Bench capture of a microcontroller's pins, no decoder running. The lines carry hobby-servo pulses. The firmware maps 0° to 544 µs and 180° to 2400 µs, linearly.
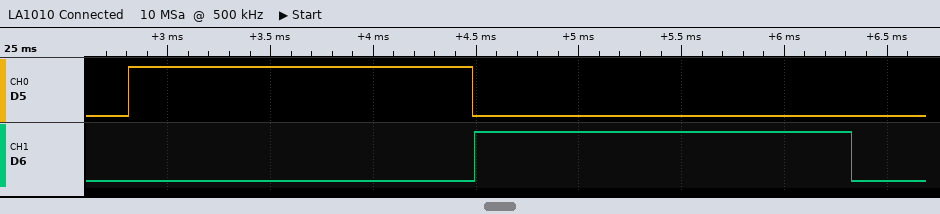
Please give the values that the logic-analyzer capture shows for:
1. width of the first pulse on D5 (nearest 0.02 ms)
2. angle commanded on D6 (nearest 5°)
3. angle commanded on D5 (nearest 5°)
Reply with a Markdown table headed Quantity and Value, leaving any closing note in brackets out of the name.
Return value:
| Quantity | Value |
|---|---|
| width of the first pulse on D5 | 1.68 ms |
| angle commanded on D6 | 125° |
| angle commanded on D5 | 110° |
